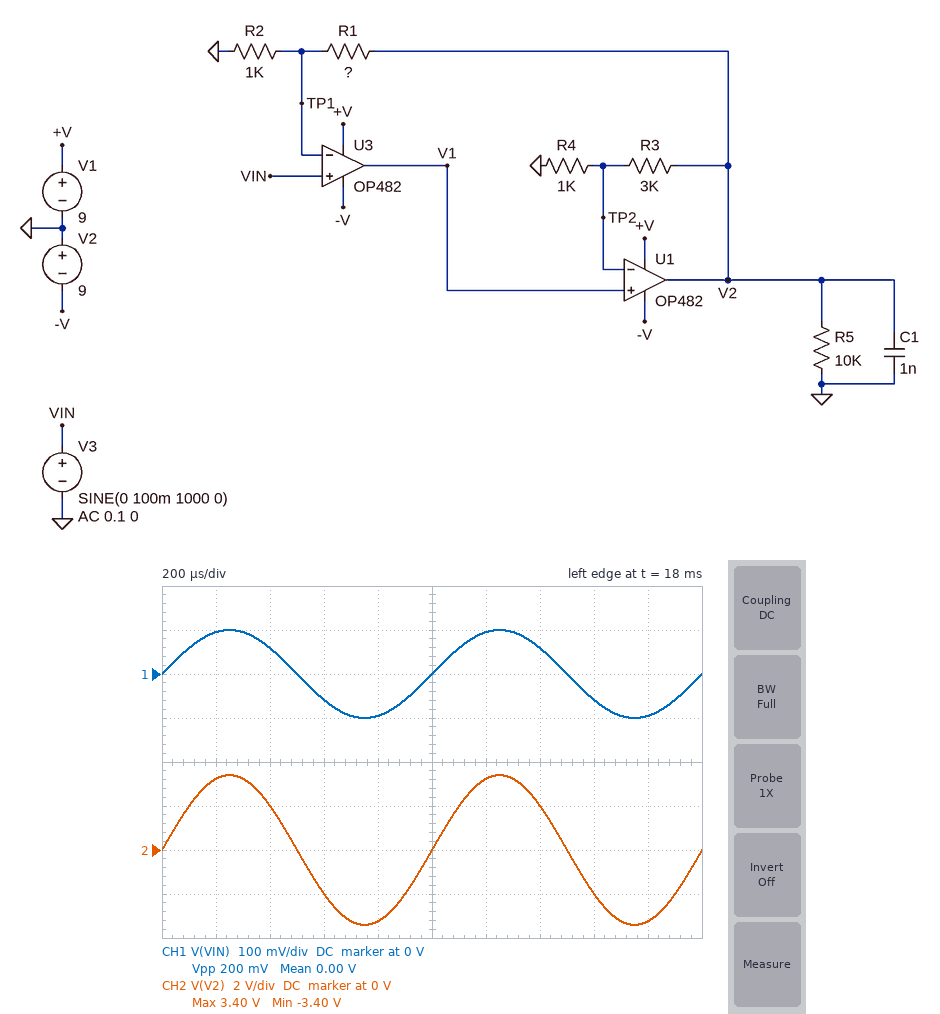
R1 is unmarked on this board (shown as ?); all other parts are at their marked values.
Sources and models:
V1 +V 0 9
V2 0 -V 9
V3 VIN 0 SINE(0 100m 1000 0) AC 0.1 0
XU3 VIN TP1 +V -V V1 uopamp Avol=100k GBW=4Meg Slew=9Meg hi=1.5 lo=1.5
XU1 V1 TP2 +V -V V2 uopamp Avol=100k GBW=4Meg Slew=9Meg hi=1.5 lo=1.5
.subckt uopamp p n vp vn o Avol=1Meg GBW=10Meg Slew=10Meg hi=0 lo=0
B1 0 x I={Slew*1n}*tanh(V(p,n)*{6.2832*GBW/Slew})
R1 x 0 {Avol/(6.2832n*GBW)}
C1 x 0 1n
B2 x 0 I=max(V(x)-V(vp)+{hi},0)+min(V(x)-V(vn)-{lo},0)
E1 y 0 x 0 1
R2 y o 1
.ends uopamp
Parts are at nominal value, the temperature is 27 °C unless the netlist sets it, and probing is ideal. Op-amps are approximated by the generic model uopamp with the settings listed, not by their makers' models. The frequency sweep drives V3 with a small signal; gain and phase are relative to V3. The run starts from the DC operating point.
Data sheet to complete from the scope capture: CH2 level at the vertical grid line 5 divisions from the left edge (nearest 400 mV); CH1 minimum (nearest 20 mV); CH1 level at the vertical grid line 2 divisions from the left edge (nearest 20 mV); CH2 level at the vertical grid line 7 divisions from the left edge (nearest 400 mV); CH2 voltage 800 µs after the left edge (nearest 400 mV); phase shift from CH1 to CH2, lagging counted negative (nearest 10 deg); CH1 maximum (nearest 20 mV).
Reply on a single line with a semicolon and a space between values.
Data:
0 V; -100 mV; 60 mV; 2.0 V; -3.2 V; 0 deg; 100 mV
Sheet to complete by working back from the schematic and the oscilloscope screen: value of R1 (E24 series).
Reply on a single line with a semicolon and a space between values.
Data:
33 kΩ
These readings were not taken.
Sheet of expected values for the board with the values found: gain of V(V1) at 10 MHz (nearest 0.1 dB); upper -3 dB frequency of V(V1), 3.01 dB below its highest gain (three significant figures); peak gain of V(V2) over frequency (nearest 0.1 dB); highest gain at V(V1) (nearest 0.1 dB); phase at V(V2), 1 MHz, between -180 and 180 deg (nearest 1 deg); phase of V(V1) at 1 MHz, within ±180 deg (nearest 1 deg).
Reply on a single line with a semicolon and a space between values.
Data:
-7.9 dB; 826 kHz; 30.6 dB; 18.7 dB; -118 deg; -73 deg
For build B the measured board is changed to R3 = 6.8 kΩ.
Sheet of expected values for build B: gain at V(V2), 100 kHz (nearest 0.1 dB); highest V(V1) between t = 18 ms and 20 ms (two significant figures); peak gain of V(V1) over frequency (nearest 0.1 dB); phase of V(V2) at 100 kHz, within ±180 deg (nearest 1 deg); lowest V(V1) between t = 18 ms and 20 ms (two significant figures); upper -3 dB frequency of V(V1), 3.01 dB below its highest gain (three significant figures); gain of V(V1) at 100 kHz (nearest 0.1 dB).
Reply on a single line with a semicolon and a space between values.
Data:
30.8 dB; 440 mV; 19.9 dB; -6 deg; -440 mV; 923 kHz; 13.1 dB
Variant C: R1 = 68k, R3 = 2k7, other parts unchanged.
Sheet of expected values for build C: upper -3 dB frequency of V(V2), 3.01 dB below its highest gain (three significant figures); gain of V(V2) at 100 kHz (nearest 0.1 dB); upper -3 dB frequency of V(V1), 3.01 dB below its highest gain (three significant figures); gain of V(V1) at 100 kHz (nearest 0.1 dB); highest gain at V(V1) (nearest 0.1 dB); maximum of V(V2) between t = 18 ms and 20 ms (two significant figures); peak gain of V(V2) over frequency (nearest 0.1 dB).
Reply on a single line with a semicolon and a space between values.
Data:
264 kHz; 36.2 dB; 279 kHz; 24.9 dB; 25.4 dB; 6.9 V; 36.8 dB
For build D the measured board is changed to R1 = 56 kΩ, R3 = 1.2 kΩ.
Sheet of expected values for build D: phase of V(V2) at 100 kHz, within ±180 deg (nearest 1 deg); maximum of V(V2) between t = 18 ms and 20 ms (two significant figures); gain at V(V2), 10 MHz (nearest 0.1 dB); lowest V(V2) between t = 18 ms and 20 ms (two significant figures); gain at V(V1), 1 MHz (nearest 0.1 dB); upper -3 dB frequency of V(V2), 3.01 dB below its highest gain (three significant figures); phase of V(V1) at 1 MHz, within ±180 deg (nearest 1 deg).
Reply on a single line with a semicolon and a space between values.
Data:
-34 deg; 5.7 V; -16.0 dB; -5.7 V; 12.6 dB; 169 kHz; -83 deg
